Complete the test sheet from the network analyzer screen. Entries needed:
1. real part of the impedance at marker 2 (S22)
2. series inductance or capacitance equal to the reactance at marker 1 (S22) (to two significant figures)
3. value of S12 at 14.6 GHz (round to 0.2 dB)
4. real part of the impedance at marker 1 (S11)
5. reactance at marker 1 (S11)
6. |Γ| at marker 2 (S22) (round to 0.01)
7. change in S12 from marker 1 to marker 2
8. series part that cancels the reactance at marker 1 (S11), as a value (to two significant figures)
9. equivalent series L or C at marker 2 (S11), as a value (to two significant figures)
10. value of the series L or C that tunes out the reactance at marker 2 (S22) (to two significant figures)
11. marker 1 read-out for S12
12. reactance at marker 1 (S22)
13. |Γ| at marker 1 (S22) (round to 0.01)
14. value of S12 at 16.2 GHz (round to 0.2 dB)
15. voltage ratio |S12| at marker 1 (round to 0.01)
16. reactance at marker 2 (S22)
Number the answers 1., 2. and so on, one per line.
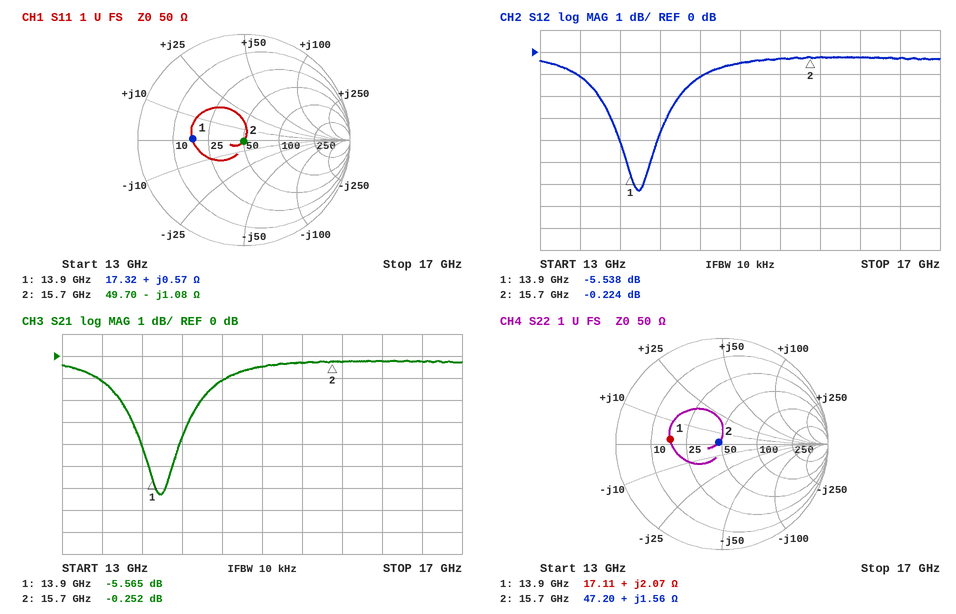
1. 47.20 Ω
2. 24 pH
3. -1.2 dB
4. 17.32 Ω
5. +0.57 Ω
6. 0.03
7. 5.314 dB
8. 20 pF
9. 9.4 pF
10. 6.5 pF
11. -5.538 dB
12. +2.07 Ω
13. 0.49
14. -0.2 dB
15. 0.53
16. +1.56 Ω
